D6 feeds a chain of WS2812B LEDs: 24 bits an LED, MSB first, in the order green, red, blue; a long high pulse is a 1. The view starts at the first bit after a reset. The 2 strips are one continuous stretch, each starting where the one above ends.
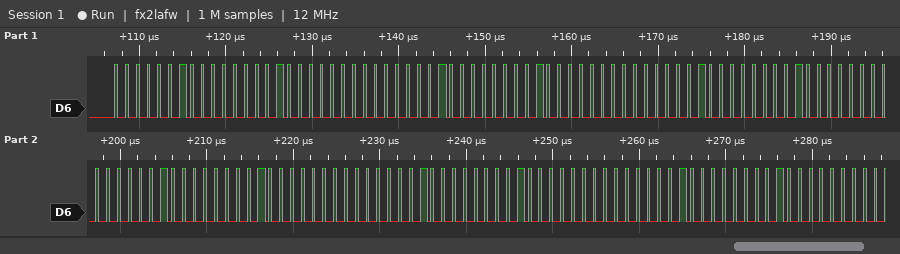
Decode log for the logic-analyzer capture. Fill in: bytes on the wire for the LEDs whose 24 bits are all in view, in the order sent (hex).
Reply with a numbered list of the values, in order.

1. 02 01 00 02 01 00 02 01 00 02 01 00 02 01 00 02 01 00
